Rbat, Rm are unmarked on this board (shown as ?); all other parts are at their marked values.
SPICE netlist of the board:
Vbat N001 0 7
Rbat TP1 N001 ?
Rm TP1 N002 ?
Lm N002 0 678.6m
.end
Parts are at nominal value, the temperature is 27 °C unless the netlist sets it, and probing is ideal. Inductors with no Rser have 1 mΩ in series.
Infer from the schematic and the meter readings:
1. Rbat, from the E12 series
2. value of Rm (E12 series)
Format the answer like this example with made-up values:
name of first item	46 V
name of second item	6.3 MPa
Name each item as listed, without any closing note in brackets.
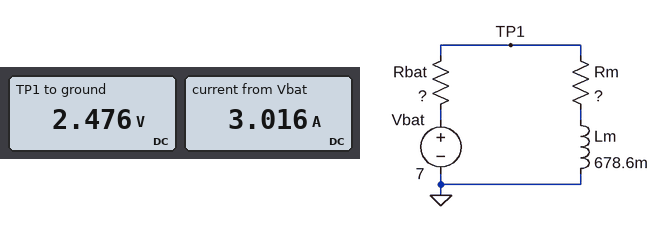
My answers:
Rbat, from the E12 series	1.5 Ω
value of Rm	0.82 Ω
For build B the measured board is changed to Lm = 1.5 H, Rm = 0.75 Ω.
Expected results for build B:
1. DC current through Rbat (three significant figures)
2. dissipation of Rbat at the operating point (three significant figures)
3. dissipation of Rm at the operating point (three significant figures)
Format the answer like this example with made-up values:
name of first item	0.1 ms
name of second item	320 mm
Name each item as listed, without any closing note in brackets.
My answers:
DC current through Rbat	3.11 A
dissipation of Rbat at the operating point	14.5 W
dissipation of Rm at the operating point	7.25 W
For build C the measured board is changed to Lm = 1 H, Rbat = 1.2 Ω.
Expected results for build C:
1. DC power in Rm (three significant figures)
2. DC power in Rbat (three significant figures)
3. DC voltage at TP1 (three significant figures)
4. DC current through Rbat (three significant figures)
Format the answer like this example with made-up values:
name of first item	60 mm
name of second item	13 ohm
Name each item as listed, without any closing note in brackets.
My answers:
DC power in Rm	9.84 W
DC power in Rbat	14.4 W
DC voltage at TP1	2.84 V
DC current through Rbat	3.46 A
